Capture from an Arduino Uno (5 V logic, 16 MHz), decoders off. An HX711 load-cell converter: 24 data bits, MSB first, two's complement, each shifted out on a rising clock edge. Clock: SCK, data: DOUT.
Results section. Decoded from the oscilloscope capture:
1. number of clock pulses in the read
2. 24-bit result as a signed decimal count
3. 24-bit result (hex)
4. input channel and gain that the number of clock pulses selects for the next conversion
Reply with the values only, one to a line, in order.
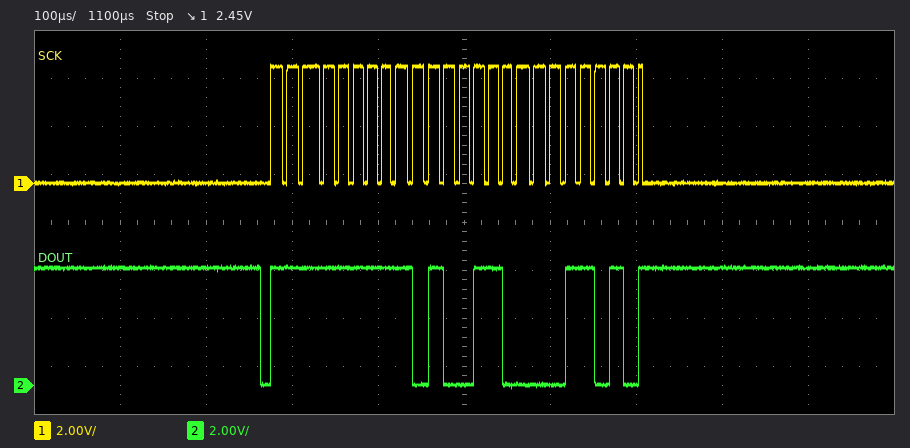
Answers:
25
-23014
0xFFA61A
channel A, gain 128
